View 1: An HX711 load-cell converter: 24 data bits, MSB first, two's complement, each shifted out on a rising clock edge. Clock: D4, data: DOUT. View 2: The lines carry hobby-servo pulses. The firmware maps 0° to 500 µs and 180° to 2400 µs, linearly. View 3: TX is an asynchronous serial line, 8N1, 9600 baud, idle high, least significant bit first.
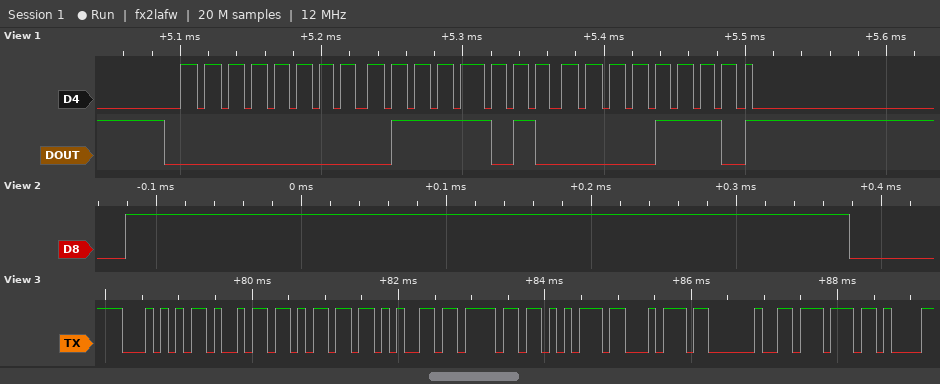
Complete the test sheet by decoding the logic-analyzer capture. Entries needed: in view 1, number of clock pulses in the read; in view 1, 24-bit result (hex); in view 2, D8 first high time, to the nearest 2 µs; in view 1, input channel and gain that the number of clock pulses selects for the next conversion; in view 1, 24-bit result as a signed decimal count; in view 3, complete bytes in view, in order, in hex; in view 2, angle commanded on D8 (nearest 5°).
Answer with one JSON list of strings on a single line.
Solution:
["25", "0x007A0E", "500 µs", "channel A, gain 128", "31246", "0x54 0x69 0x6D 0x65 0x6F 0x75 0x74 0x20 0x77", "0°"]
